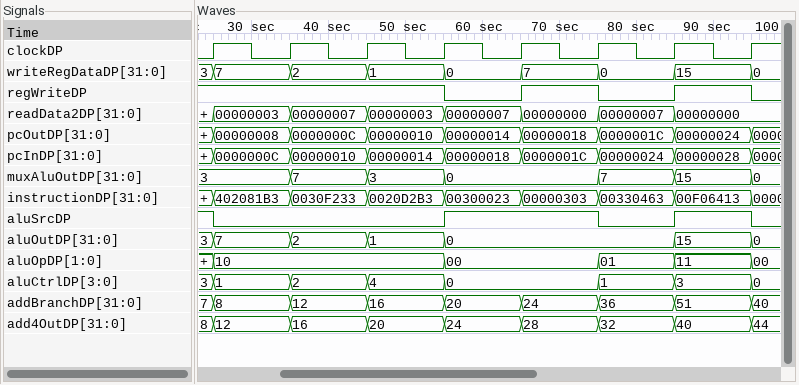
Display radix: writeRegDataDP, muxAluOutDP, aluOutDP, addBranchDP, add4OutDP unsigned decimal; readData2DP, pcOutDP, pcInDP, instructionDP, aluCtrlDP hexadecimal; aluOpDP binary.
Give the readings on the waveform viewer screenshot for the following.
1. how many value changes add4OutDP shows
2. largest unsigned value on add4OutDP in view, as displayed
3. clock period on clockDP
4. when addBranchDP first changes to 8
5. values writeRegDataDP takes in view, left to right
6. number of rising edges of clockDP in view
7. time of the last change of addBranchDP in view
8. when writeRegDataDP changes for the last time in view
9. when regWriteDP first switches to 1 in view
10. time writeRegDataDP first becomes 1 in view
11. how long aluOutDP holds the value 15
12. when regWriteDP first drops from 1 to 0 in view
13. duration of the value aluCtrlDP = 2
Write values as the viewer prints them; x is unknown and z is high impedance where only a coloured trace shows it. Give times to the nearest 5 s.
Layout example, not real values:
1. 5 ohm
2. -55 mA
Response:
1. 8
2. 44
3. 10 s
4. 25 s
5. 3, 7, 2, 1, 0, 7, 0, 15, 0
6. 8
7. 95 s
8. 95 s
9. 65 s
10. 45 s
11. 10 s
12. 55 s
13. 10 s
